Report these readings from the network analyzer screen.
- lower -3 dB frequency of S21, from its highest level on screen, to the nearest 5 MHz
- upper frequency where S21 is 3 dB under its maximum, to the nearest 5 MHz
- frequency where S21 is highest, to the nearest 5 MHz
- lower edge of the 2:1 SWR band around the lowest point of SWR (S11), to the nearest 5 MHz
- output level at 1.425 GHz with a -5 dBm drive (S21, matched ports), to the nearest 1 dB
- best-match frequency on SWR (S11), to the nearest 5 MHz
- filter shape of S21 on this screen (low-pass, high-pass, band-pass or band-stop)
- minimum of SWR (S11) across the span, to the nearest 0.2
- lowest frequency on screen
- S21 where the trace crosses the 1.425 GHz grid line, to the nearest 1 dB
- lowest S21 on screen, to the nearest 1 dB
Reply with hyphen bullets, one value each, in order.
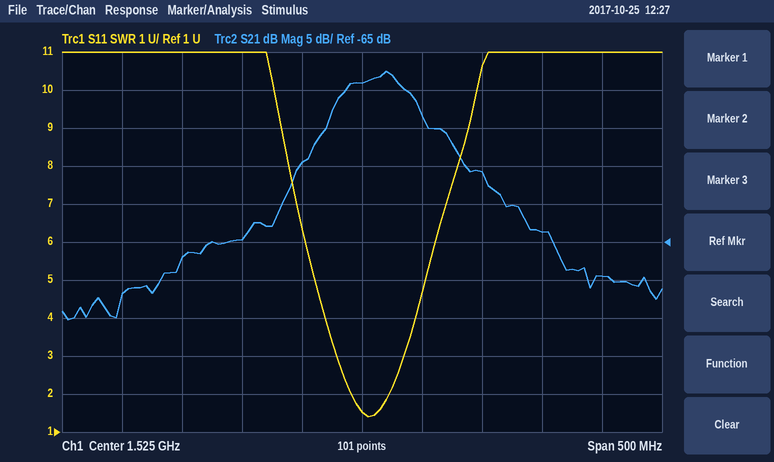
- 1.510 GHz
- 1.565 GHz
- 1.545 GHz
- 1.515 GHz
- -70 dBm
- 1.530 GHz
- band-pass
- 1.4
- 1.275 GHz
- -65 dB
- -75 dB
